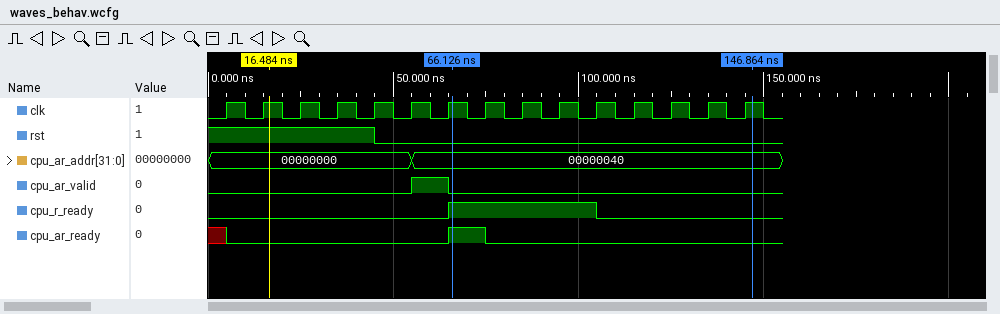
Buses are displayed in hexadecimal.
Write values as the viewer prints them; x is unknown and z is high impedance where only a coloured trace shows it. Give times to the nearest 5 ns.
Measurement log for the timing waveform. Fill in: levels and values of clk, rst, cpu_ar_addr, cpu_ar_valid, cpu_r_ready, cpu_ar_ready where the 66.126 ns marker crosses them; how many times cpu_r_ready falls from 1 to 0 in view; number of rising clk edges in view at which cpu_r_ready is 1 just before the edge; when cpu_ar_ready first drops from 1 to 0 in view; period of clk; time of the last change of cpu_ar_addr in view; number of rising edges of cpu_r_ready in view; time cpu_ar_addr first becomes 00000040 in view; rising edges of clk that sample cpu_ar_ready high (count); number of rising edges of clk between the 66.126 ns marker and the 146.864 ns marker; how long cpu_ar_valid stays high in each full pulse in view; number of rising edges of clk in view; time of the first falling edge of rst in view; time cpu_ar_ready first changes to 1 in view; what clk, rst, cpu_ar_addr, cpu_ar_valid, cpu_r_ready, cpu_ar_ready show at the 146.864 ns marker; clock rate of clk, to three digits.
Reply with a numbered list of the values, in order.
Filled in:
1. clk=1, rst=0, cpu_ar_addr=00000040, cpu_ar_valid=0, cpu_r_ready=1, cpu_ar_ready=1
2. 1
3. 4
4. 75 ns
5. 10 ns
6. 55 ns
7. 1
8. 55 ns
9. 1
10. 8
11. 10 ns
12. 15
13. 45 ns
14. 65 ns
15. clk=1, rst=0, cpu_ar_addr=00000040, cpu_ar_valid=0, cpu_r_ready=0, cpu_ar_ready=0
16. 100 MHz
